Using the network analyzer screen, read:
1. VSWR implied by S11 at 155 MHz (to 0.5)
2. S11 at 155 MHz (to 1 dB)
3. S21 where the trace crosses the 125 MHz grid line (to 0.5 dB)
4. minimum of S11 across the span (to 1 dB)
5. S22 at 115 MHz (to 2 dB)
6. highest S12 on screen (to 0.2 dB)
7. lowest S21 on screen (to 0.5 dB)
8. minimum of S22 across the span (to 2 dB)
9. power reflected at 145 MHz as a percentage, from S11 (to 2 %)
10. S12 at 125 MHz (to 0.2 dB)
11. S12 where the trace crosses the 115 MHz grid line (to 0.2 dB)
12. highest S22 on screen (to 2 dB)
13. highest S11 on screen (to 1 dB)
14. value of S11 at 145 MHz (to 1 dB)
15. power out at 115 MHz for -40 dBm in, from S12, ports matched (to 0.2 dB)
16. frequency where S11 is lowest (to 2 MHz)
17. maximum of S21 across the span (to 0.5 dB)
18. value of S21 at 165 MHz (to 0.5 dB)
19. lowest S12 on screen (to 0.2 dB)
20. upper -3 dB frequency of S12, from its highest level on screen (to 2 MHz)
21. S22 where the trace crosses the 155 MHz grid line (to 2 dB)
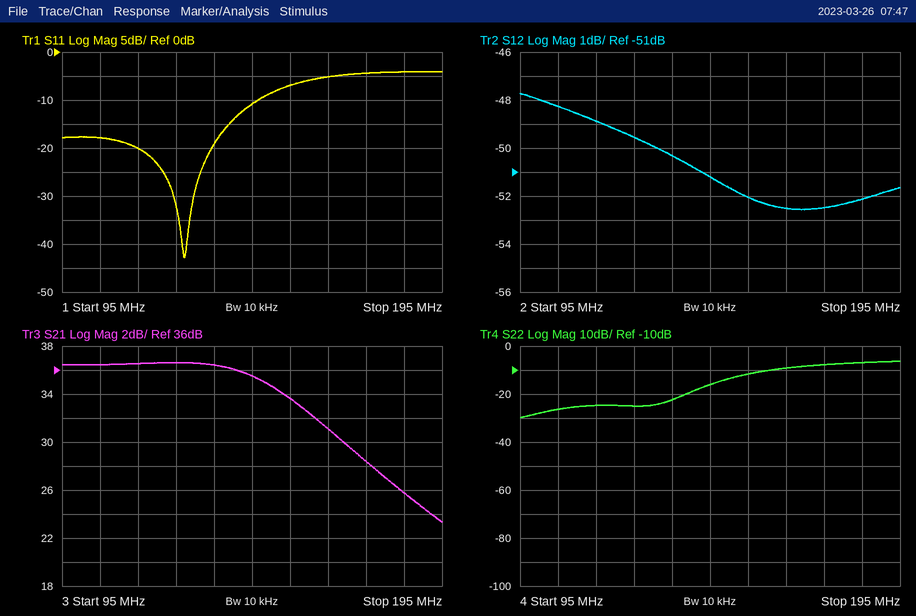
2.5
-7 dB
36.5 dB
-43 dB
-24 dB
-47.8 dB
23.5 dB
-30 dB
8 %
-49.6 dB
-48.8 dB
-6 dB
-4 dB
-11 dB
-88.8 dBm
128 MHz
36.5 dB
31.0 dB
-52.6 dB
140 MHz
-12 dB
